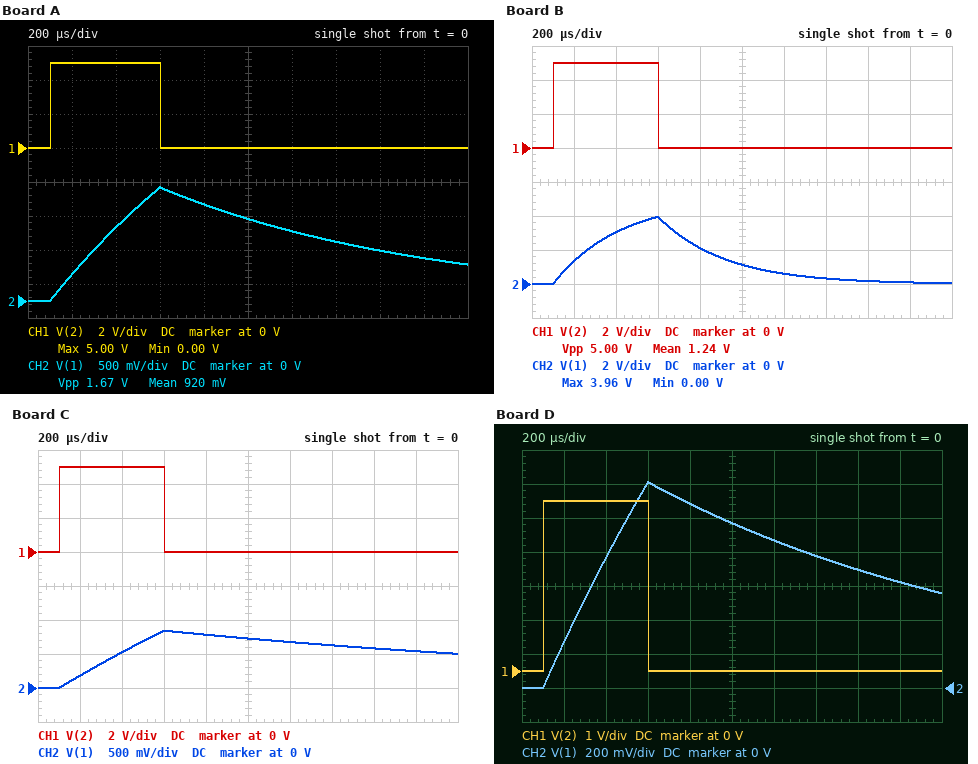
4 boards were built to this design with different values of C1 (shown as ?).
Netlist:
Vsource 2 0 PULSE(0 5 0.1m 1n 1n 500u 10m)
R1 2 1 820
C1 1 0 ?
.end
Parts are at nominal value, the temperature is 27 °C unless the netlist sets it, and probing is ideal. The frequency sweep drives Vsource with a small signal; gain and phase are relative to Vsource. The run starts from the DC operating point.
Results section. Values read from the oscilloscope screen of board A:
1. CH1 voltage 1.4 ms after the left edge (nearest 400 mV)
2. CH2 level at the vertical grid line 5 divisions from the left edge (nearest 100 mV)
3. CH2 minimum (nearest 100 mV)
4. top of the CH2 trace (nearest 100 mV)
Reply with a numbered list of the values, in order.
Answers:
1. 0 V
2. 1.2 V
3. 0 V
4. 1.7 V
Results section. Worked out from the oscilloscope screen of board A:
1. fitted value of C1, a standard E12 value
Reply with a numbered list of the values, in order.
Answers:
1. 1.5 µF
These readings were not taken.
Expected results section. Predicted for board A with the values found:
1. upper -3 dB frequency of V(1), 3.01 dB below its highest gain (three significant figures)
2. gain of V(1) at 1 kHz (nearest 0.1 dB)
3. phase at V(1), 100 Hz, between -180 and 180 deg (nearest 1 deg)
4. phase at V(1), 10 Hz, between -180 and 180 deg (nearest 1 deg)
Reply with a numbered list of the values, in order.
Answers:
1. 129 Hz
2. -17.8 dB
3. -38 deg
4. -4 deg
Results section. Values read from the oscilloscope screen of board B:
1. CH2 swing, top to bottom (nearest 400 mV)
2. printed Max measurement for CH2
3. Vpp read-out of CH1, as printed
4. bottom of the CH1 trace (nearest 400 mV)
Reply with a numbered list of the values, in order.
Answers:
1. 4.0 V
2. 3.96 V
3. 5.00 V
4. 0 V
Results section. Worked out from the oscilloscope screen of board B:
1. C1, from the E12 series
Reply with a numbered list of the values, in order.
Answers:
1. 390 nF
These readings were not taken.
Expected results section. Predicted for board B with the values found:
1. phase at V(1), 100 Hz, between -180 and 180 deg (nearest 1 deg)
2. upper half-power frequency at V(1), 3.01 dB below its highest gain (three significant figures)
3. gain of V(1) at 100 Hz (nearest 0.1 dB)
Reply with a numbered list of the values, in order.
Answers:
1. -11 deg
2. 498 Hz
3. -0.2 dB
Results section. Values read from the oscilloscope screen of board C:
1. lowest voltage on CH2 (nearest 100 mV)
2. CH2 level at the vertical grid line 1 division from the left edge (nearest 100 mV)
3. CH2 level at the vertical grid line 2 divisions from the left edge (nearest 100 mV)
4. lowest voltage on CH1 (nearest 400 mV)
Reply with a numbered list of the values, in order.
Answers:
1. 0 V
2. 200 mV
3. 500 mV
4. 0 V
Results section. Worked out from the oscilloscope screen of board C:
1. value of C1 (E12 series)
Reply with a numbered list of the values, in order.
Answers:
1. 3.3 µF
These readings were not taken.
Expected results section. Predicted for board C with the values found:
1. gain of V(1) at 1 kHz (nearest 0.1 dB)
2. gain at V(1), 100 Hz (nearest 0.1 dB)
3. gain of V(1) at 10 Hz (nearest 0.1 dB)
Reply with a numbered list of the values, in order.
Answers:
1. -24.6 dB
2. -5.9 dB
3. -0.1 dB
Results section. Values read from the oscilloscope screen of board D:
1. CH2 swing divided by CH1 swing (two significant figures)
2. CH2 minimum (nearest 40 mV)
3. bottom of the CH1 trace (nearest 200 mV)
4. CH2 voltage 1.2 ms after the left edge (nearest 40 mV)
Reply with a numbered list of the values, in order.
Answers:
1. 0.24
2. 0 V
3. 0 V
4. 880 mV
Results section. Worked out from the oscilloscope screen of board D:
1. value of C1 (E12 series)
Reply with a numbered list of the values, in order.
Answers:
1. 2.2 µF
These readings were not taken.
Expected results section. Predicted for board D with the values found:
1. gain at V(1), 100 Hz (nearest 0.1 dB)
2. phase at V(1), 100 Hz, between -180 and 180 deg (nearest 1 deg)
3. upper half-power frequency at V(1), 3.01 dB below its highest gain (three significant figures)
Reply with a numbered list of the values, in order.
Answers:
1. -3.6 dB
2. -49 deg
3. 88.2 Hz
